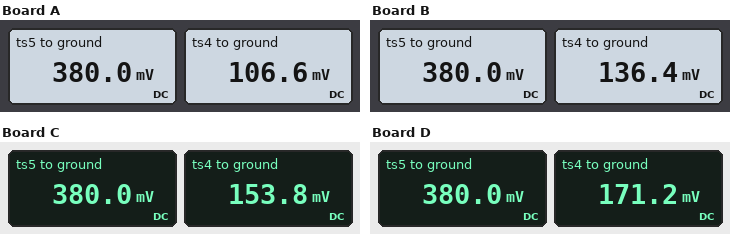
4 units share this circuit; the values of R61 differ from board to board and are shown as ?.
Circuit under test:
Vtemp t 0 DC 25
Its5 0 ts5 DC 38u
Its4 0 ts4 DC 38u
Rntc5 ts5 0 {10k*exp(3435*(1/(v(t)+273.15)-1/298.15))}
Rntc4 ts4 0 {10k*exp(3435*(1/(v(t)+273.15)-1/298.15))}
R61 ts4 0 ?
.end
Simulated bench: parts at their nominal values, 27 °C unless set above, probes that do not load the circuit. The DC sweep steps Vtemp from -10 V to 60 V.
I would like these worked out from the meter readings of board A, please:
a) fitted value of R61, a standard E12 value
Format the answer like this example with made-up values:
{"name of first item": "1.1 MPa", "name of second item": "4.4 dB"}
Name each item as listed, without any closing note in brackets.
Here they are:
{"fitted value of R61, a standard E12 value": "3.9 kΩ"}
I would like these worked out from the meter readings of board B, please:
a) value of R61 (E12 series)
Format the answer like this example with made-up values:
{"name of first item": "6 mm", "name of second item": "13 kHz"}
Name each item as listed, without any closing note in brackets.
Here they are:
{"value of R61": "5.6 kΩ"}
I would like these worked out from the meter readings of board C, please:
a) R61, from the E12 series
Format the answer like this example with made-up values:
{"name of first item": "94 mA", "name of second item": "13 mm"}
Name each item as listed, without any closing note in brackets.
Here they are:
{"R61, from the E12 series": "6.8 kΩ"}
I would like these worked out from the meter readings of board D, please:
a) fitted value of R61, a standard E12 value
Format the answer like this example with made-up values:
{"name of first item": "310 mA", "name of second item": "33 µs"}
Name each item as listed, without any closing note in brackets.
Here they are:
{"fitted value of R61, a standard E12 value": "8.2 kΩ"}
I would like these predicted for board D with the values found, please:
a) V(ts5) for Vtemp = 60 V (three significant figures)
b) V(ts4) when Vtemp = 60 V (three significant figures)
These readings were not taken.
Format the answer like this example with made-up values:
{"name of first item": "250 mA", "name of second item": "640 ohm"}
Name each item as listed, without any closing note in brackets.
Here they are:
{"V(ts5) for Vtemp = 60 V": "113 mV", "V(ts4) when Vtemp = 60 V": "83.1 mV"}
